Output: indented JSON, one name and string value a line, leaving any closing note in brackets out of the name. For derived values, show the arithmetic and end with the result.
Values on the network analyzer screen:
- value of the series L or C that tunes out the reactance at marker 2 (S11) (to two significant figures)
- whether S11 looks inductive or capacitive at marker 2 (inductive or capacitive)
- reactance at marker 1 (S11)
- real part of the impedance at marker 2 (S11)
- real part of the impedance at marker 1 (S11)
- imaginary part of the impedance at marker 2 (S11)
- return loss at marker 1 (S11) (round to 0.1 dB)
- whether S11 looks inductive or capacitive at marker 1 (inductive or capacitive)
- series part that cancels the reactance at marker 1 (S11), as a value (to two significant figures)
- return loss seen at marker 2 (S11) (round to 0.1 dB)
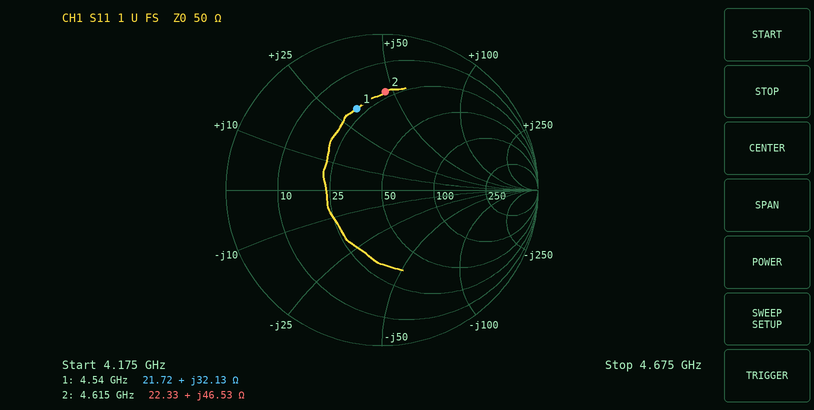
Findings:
{
  "value of the series L or C that tunes out the reactance at marker 2 (S11)": "C = 1/(2π × 4.615 GHz × 46.53 Ω) ≈ 741 fF, so 740 fF to two significant figures",
  "whether S11 looks inductive or capacitive at marker 2": "inductive",
  "reactance at marker 1": "+32.13 Ω",
  "real part of the impedance at marker 2": "22.33 Ω",
  "real part of the impedance at marker 1": "21.72 Ω",
  "imaginary part of the impedance at marker 2": "+46.53 Ω",
  "return loss at marker 1 (S11)": "5.3 dB",
  "whether S11 looks inductive or capacitive at marker 1": "inductive",
  "series part that cancels the reactance at marker 1 (S11), as a value": "C = 1/(2π × 4.54 GHz × 32.13 Ω) ≈ 1.1 pF",
  "return loss seen at marker 2 (S11)": "4.0 dB"
}
